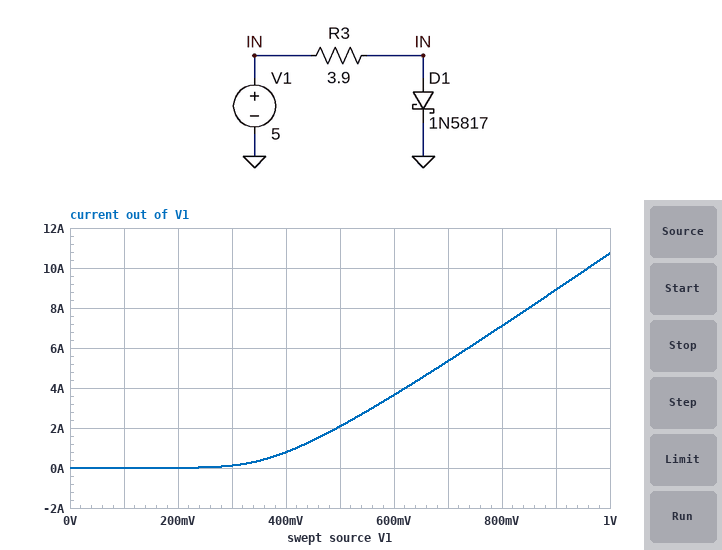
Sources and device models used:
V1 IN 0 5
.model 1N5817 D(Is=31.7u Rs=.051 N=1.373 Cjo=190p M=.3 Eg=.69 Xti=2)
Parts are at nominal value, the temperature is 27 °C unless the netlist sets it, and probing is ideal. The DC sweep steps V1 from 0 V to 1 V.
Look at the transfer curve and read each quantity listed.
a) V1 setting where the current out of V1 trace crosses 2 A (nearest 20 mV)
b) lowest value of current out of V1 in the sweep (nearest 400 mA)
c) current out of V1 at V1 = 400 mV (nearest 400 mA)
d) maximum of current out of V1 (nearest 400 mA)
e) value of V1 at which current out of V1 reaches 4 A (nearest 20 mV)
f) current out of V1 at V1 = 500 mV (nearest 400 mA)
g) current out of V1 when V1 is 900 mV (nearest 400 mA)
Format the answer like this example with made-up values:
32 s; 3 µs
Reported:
500 mV; 0 A; 800 mA; 10.8 A; 620 mV; 2.0 A; 8.8 A
